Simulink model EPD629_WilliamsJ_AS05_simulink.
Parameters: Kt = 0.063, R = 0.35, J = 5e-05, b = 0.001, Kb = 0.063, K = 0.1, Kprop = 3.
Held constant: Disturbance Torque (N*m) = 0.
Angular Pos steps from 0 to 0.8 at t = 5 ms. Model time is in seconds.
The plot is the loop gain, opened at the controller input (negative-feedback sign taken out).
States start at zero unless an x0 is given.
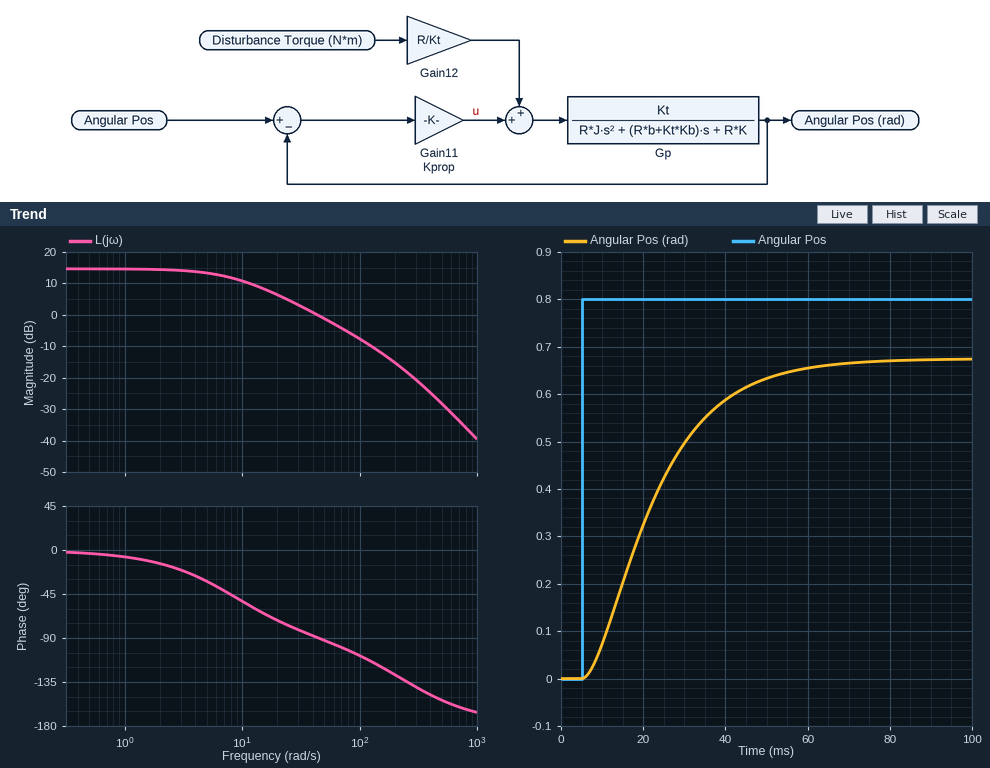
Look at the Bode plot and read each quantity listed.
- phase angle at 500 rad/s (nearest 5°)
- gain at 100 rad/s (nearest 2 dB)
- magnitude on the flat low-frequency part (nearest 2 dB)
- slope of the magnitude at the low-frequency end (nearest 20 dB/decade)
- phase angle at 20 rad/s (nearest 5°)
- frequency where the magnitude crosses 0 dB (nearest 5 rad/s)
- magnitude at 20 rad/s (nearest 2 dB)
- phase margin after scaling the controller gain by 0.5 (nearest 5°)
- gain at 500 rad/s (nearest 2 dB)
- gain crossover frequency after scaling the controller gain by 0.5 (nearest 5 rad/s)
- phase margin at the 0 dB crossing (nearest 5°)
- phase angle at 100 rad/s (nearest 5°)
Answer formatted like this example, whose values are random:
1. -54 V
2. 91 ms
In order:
1. -155°
2. -8 dB
3. 14 dB
4. 0 dB/decade
5. -70°
6. 45 rad/s
7. 6 dB
8. 105°
9. -28 dB
10. 20 rad/s
11. 90°
12. -110°
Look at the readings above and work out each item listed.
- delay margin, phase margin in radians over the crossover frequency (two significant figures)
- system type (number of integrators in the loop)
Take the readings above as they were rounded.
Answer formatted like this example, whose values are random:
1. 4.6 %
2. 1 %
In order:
1. 0.035 s
2. 0
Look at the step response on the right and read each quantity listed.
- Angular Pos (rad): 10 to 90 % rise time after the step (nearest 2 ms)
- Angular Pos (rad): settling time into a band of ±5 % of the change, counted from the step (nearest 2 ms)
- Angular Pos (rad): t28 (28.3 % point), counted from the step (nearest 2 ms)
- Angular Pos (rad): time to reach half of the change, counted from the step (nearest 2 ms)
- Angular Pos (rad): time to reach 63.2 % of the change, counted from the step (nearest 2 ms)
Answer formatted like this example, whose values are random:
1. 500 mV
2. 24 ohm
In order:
1. 34 ms
2. 48 ms
3. 10 ms
4. 16 ms
5. 20 ms
